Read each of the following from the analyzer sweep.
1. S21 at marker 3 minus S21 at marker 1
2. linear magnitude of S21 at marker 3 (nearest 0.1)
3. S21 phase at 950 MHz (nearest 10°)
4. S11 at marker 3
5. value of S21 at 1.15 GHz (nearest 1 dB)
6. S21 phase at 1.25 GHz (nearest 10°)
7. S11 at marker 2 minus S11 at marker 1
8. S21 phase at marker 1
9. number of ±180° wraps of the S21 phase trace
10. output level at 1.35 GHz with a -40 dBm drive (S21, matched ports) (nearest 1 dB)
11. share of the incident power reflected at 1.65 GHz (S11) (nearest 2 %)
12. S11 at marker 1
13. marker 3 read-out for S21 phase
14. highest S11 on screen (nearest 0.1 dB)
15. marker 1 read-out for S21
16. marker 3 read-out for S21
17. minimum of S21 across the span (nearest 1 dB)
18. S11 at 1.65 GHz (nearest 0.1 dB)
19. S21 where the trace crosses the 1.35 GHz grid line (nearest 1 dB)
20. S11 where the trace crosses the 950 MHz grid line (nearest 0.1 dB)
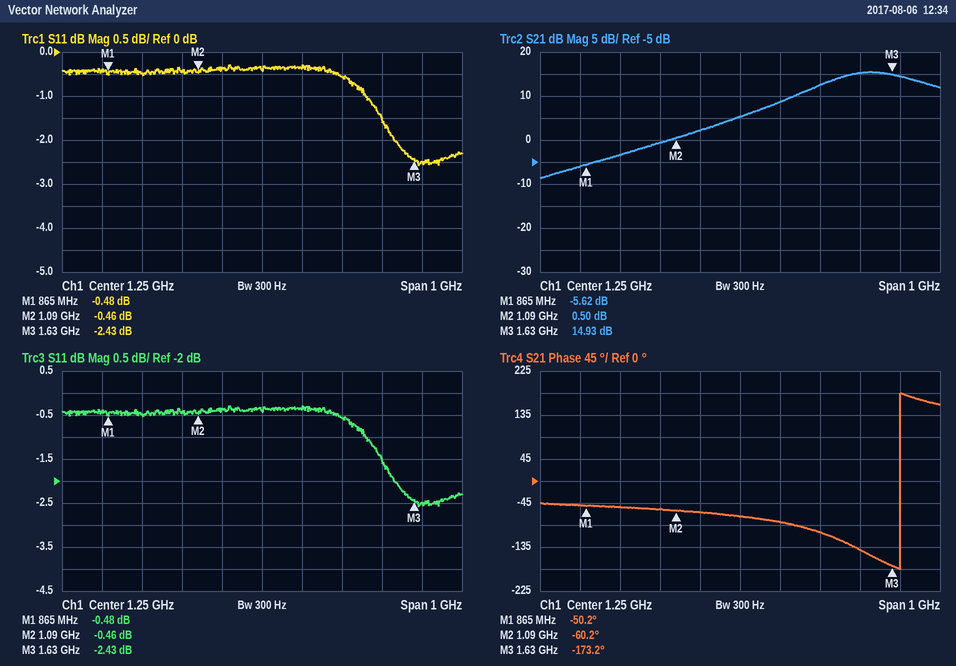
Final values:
20.55 dB
5.6
-50°
-2.43 dB
2 dB
-70°
0.02 dB
-50.2°
1
-31 dBm
56 %
-0.48 dB
-173.2°
-0.3 dB
-5.62 dB
14.93 dB
-9 dB
-2.5 dB
9 dB
-0.5 dB
